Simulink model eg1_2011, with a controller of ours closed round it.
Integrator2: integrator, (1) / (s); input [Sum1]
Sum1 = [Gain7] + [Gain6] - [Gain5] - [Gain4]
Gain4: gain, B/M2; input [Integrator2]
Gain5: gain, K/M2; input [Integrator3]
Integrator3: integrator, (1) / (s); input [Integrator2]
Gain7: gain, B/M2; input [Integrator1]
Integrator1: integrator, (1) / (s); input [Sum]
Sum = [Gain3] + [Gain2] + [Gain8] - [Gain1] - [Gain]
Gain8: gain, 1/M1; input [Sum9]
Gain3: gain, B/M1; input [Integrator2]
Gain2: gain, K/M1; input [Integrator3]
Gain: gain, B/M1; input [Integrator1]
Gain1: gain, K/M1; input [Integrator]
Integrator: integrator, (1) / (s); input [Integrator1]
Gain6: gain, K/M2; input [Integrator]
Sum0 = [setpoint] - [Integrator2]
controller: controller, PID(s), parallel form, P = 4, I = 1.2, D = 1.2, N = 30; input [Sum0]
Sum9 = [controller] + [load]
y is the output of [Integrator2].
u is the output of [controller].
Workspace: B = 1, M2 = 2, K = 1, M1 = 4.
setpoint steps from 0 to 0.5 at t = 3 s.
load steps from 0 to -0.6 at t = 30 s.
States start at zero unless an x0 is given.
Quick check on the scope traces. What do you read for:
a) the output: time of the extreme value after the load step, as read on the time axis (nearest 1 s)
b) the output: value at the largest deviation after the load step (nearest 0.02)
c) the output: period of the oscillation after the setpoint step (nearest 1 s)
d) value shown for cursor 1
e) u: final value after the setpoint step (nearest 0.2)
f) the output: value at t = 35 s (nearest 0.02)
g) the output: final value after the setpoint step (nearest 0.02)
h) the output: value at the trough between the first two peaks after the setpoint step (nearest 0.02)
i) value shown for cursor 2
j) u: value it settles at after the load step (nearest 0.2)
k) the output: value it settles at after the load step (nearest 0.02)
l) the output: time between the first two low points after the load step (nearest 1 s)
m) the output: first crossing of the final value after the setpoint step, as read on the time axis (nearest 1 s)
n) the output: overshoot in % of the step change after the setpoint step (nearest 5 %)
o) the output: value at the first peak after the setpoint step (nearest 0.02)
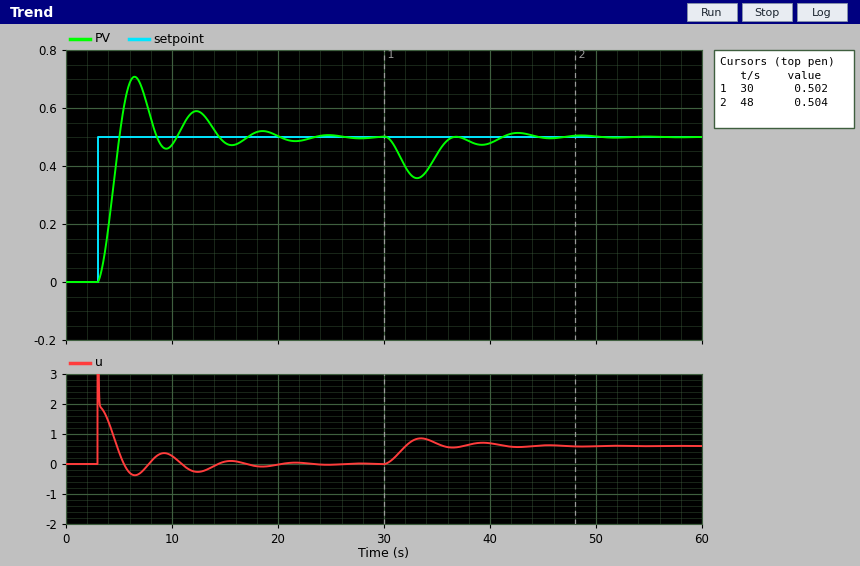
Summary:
33 s
0.36
6 s
0.502
0.0
0.44
0.50
0.46
0.504
0.6
0.50
6 s
5 s
40 %
0.70
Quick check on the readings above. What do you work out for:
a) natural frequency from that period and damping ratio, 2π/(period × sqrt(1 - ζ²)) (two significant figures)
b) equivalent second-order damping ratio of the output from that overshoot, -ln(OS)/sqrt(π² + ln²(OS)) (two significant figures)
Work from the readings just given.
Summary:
1.1 rad/s
0.28
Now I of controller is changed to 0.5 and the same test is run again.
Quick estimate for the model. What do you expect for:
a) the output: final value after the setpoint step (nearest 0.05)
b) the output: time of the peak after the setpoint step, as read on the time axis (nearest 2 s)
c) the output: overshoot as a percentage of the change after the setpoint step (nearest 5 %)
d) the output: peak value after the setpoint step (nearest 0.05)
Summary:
0.50
6 s
25 %
0.60
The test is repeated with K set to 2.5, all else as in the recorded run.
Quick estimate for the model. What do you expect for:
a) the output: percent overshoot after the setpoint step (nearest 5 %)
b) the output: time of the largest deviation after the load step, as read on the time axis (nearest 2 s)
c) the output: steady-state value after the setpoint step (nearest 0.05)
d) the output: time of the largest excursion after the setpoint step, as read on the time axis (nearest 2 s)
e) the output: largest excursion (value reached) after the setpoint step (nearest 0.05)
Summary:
30 %
32 s
0.50
10 s
0.65
